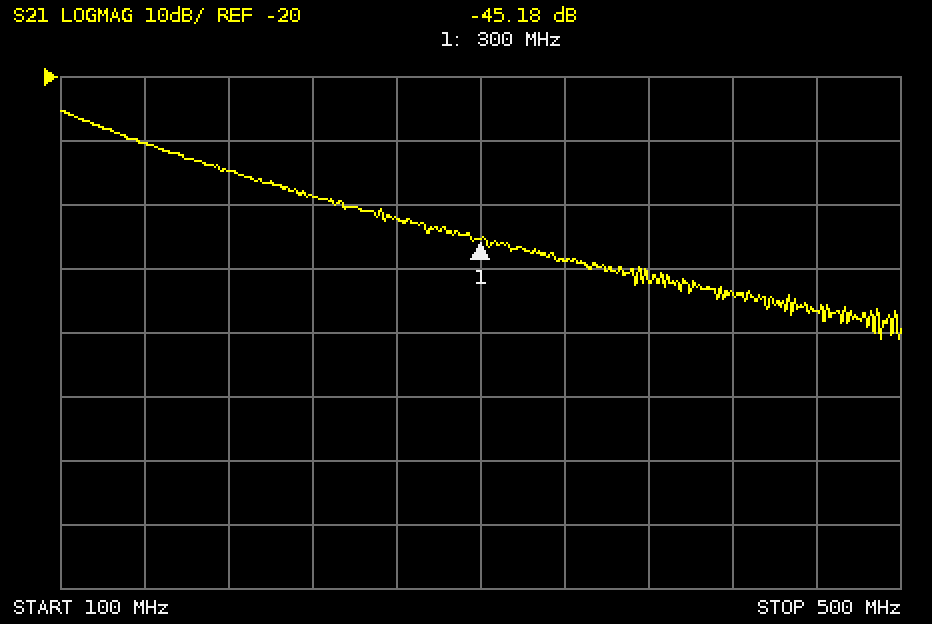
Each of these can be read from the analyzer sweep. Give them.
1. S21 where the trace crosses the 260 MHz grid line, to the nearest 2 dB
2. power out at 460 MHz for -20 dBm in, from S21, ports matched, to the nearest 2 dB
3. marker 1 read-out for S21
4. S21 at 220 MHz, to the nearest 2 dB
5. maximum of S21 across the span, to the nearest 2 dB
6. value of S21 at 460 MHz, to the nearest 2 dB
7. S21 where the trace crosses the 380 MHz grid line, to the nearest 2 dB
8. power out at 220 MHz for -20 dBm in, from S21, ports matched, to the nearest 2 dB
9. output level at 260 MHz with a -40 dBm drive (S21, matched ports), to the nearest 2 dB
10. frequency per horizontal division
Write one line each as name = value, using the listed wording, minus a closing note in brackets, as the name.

S21 where the trace crosses the 260 MHz grid line, to the nearest 2 dB = -42 dB
power out at 460 MHz for -20 dBm in, from S21, ports matched, to the nearest 2 dB = -76 dBm
marker 1 read-out for S21 = -45.18 dB
S21 at 220 MHz, to the nearest 2 dB = -38 dB
maximum of S21 across the span, to the nearest 2 dB = -26 dB
value of S21 at 460 MHz, to the nearest 2 dB = -56 dB
S21 where the trace crosses the 380 MHz grid line, to the nearest 2 dB = -52 dB
power out at 220 MHz for -20 dBm in, from S21, ports matched, to the nearest 2 dB = -58 dBm
output level at 260 MHz with a -40 dBm drive (S21, matched ports), to the nearest 2 dB = -82 dBm
frequency per horizontal division = 40 MHz
